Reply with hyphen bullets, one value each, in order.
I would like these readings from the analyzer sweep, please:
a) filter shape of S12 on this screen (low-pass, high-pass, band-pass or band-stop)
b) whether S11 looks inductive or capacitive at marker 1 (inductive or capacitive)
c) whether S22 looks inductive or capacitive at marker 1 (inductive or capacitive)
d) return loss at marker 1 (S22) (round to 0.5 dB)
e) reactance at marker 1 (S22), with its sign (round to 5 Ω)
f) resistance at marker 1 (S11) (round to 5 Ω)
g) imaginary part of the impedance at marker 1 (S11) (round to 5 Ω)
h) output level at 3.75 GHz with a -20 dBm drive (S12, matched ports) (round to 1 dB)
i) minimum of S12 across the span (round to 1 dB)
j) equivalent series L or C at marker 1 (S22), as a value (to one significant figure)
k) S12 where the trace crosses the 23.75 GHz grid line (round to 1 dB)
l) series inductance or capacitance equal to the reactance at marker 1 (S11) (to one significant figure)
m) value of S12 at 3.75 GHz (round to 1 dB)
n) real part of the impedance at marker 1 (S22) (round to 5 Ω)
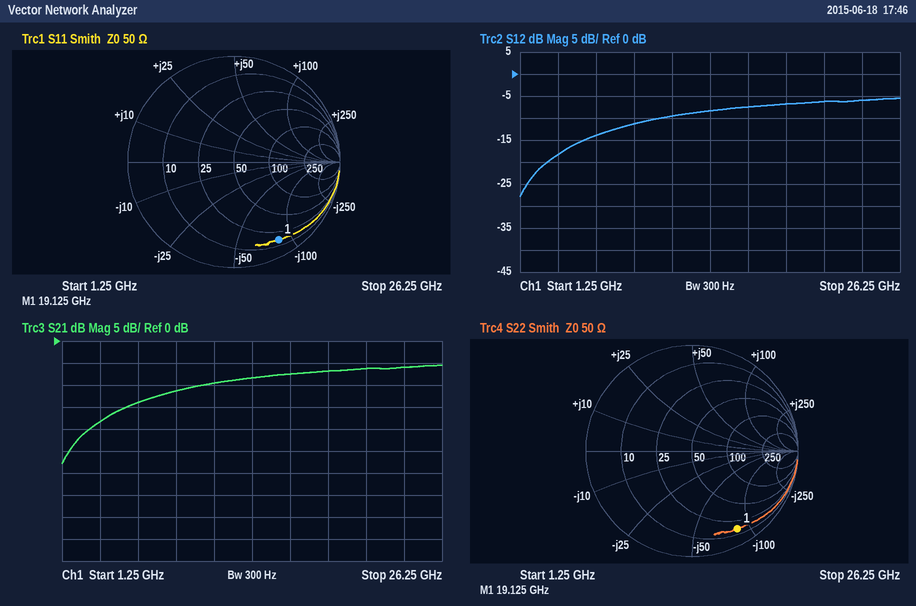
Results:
- high-pass
- capacitive
- capacitive
- 1.5 dB
- -85 Ω
- 15 Ω
- -85 Ω
- -38 dBm
- -28 dB
- 100 fF
- -6 dB
- 100 fF
- -18 dB
- 15 Ω
